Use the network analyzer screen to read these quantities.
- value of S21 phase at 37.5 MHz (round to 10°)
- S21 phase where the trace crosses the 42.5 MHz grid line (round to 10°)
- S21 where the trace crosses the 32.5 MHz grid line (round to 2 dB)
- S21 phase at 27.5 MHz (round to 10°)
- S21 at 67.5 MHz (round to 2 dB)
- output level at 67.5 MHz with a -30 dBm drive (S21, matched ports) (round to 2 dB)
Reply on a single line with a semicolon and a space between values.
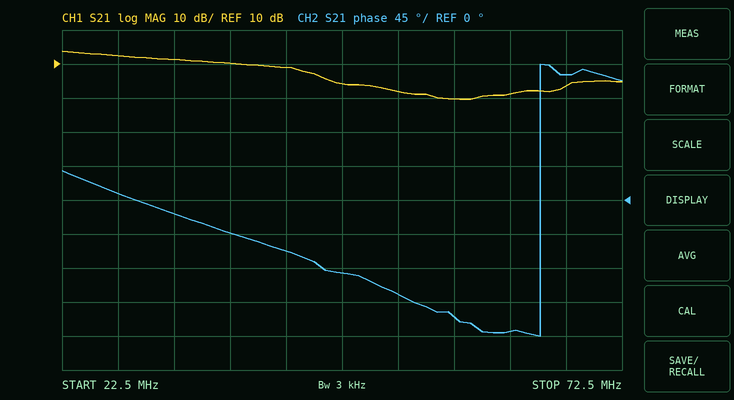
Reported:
-40°; -70°; 12 dB; 10°; 4 dB; -26 dBm
